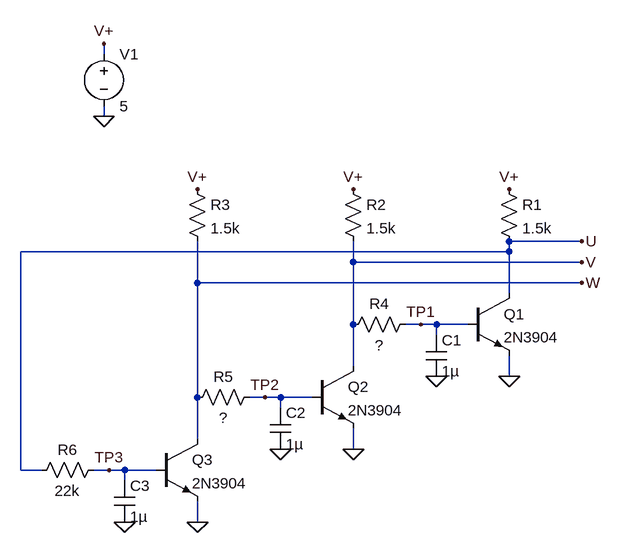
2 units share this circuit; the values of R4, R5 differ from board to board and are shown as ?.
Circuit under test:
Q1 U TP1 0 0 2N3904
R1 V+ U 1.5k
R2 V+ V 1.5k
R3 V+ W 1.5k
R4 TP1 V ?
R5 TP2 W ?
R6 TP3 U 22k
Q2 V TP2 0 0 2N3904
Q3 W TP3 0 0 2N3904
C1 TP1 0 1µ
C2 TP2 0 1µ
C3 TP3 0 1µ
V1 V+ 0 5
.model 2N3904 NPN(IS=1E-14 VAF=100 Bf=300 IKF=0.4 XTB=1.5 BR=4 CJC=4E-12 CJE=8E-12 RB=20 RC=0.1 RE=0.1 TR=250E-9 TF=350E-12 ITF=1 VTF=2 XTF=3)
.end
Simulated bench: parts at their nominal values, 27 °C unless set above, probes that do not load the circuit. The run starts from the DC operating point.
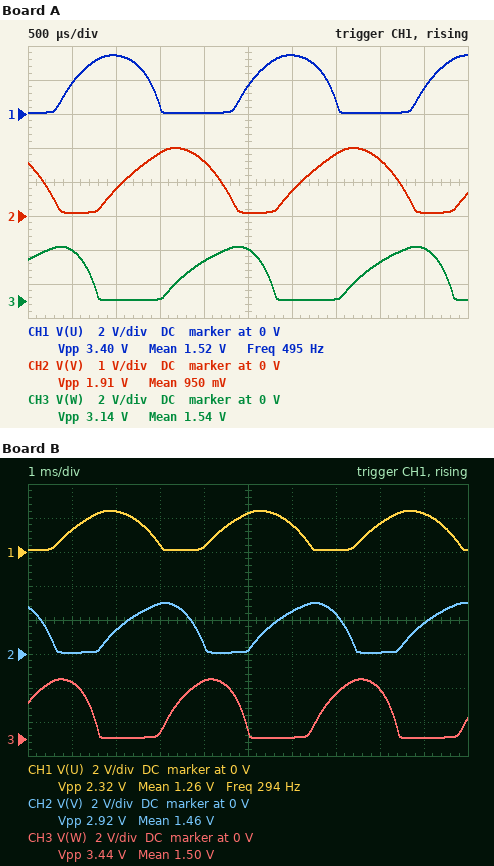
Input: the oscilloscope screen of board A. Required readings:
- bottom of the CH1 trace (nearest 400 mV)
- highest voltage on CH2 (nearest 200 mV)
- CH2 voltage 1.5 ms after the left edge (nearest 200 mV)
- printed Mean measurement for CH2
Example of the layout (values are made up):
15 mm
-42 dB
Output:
0 V
2.0 V
1.8 V
950 mV
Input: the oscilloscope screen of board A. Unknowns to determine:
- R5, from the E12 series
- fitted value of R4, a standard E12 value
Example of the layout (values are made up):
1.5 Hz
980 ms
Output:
56 kΩ
10 kΩ
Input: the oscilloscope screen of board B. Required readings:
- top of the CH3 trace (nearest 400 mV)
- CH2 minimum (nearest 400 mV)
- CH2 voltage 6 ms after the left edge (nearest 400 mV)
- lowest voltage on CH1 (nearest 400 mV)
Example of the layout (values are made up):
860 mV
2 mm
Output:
3.6 V
0 V
2.4 V
0 V
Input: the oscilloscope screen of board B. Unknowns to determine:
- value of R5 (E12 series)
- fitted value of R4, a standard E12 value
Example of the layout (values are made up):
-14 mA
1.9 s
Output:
56 kΩ
68 kΩ
